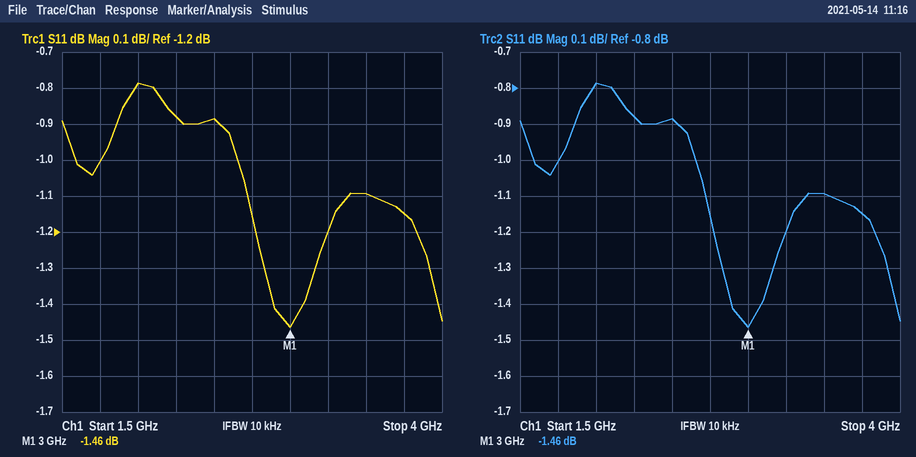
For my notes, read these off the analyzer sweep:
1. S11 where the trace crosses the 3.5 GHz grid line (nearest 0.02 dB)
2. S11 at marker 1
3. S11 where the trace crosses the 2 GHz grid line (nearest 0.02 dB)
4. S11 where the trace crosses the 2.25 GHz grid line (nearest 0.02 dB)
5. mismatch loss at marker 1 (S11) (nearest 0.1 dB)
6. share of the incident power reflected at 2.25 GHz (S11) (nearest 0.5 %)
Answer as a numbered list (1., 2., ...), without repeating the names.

1. -1.10 dB
2. -1.46 dB
3. -0.78 dB
4. -0.88 dB
5. 5.4 dB
6. 81.5 %
